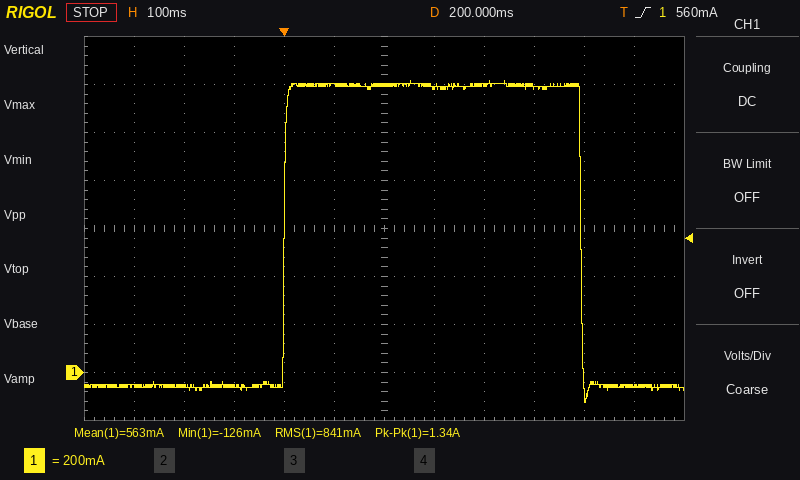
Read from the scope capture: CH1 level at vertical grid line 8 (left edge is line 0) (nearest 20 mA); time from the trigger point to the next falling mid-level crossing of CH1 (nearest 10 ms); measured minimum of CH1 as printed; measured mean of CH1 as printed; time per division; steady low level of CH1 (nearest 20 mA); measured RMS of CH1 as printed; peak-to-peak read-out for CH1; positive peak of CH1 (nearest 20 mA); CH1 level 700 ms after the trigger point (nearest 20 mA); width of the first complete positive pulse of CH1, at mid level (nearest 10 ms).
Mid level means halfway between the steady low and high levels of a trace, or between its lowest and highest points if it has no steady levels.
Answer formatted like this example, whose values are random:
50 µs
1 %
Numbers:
1.20 A
590 ms
-126 mA
563 mA
100 ms
-60 mA
841 mA
1.34 A
1.22 A
-60 mA
590 ms
